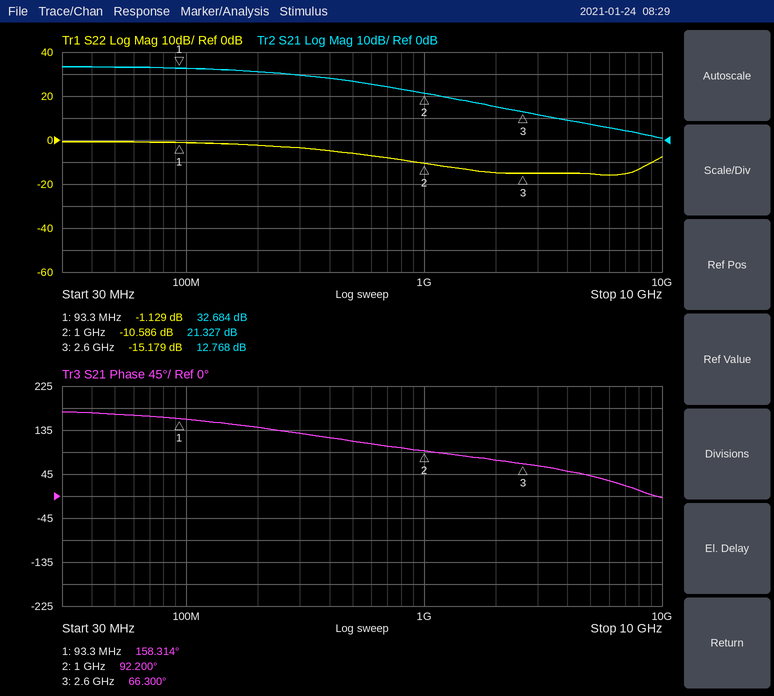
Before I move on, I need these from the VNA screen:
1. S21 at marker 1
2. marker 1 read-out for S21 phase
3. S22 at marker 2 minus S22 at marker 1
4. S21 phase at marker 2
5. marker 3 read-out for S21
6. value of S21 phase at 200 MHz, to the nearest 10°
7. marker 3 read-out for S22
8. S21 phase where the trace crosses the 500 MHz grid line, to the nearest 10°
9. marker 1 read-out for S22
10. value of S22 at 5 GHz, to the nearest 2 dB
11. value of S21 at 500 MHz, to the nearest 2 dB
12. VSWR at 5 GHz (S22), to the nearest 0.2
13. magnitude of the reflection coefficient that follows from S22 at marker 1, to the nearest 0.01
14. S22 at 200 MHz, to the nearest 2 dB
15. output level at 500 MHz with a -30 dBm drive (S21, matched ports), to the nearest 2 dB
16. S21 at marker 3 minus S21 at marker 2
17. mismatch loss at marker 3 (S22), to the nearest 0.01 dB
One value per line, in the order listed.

32.684 dB
158.314°
-9.457 dB
92.200°
12.768 dB
140°
-15.179 dB
110°
-1.129 dB
-16 dB
26 dB
1.4
0.88
-2 dB
-4 dBm
-8.559 dB
0.13 dB
